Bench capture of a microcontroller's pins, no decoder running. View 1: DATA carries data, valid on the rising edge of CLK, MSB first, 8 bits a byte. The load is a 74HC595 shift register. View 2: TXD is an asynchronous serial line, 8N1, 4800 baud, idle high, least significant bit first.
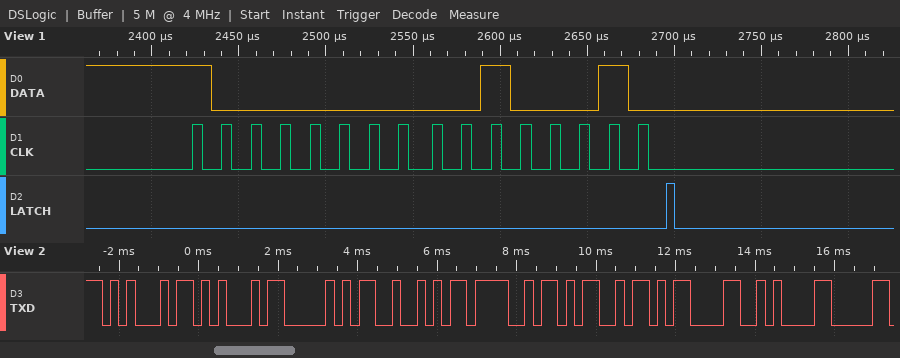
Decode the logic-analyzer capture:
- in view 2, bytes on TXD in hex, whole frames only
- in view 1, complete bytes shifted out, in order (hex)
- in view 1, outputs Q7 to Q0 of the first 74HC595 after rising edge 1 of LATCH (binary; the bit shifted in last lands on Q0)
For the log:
45 45 50 52 4F 4D 0D 0A
80 22
00100010
